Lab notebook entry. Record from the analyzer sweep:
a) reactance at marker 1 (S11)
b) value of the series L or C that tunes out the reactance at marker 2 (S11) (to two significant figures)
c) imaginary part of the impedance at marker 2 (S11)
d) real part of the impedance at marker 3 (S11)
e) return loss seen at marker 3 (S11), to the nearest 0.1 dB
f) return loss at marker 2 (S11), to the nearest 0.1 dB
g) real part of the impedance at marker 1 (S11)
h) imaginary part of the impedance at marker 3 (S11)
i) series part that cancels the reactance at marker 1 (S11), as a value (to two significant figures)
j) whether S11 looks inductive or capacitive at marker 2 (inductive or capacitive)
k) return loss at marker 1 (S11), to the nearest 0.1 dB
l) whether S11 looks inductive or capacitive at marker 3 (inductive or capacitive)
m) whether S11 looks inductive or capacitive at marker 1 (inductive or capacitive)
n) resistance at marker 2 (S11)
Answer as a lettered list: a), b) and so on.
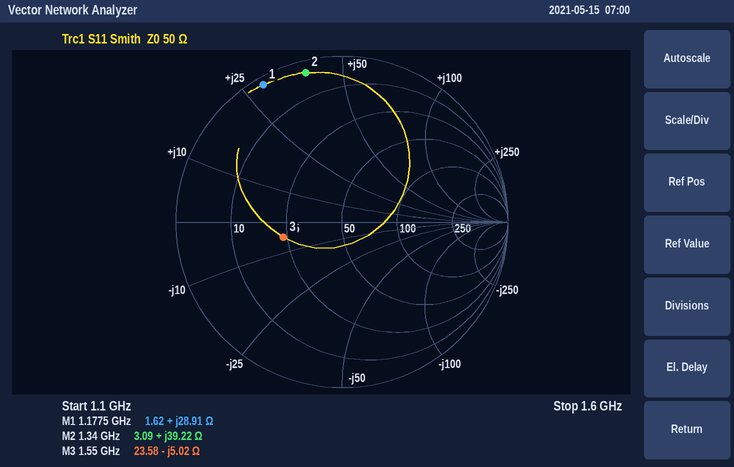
a) +28.91 Ω
b) 3.0 pF
c) +39.22 Ω
d) 23.58 Ω
e) 8.8 dB
f) 0.7 dB
g) 1.62 Ω
h) -5.02 Ω
i) 4.7 pF
j) inductive
k) 0.4 dB
l) capacitive
m) inductive
n) 3.09 Ω
